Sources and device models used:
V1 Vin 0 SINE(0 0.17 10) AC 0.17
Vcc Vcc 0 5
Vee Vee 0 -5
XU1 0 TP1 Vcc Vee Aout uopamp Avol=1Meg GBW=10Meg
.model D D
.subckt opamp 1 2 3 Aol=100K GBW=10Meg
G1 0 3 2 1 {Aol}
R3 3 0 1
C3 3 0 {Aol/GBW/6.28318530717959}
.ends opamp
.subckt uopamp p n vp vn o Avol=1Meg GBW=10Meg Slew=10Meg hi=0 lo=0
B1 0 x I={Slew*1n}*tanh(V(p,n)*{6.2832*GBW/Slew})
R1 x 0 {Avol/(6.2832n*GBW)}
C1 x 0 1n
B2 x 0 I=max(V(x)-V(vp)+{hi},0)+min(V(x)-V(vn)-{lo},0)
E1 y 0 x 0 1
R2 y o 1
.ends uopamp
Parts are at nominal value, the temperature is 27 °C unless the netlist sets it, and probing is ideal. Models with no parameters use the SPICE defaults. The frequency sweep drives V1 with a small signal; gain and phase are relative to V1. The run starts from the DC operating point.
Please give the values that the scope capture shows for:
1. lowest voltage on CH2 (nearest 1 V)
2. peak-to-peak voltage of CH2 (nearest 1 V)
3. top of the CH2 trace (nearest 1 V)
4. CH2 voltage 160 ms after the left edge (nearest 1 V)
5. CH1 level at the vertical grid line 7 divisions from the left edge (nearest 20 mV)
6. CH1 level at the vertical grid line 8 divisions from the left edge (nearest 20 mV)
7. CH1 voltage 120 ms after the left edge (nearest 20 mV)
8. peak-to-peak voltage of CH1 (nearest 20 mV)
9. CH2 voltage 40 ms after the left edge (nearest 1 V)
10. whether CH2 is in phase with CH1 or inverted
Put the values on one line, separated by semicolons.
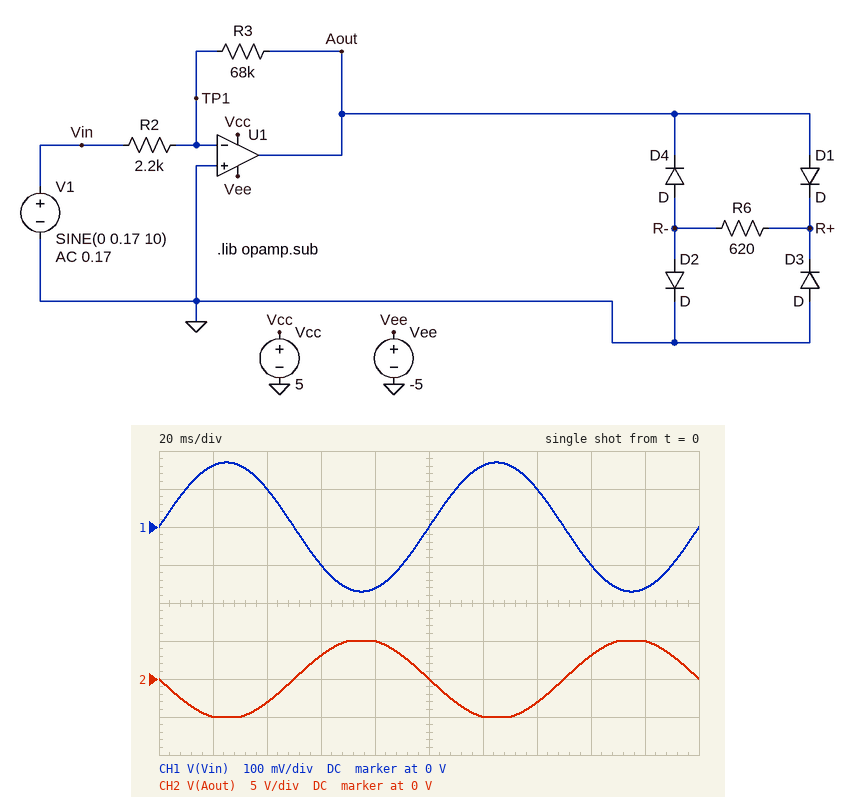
-5 V; 10 V; 5 V; 3 V; 100 mV; -100 mV; 160 mV; 340 mV; -3 V; inverted
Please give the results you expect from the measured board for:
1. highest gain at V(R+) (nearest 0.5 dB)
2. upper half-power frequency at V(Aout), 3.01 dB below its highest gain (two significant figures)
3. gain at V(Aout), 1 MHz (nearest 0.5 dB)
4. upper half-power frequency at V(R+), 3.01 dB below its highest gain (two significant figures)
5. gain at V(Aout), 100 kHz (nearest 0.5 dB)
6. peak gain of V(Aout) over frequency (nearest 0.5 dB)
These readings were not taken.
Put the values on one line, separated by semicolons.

24.0 dB; 310 kHz; 19.5 dB; 310 kHz; 29.5 dB; 30.0 dB
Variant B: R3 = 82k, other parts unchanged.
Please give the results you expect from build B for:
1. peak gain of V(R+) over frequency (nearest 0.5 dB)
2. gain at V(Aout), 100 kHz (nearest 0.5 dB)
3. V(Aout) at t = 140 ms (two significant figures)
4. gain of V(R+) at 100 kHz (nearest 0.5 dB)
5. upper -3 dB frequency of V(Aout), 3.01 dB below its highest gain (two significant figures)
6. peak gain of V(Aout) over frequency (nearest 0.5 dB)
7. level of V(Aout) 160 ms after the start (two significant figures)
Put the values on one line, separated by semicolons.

25.5 dB; 31.0 dB; -3.7 V; 25.0 dB; 260 kHz; 31.5 dB; 3.7 V
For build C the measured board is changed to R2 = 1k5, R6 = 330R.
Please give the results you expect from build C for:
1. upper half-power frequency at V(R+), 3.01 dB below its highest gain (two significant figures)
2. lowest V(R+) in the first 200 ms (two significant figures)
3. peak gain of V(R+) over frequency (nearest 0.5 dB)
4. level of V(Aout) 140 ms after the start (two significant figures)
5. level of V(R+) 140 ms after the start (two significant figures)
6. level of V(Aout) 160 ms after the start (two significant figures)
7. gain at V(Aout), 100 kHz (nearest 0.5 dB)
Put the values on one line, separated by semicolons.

220 kHz; -720 mV; 27.0 dB; -4.5 V; -710 mV; 4.5 V; 32.5 dB
